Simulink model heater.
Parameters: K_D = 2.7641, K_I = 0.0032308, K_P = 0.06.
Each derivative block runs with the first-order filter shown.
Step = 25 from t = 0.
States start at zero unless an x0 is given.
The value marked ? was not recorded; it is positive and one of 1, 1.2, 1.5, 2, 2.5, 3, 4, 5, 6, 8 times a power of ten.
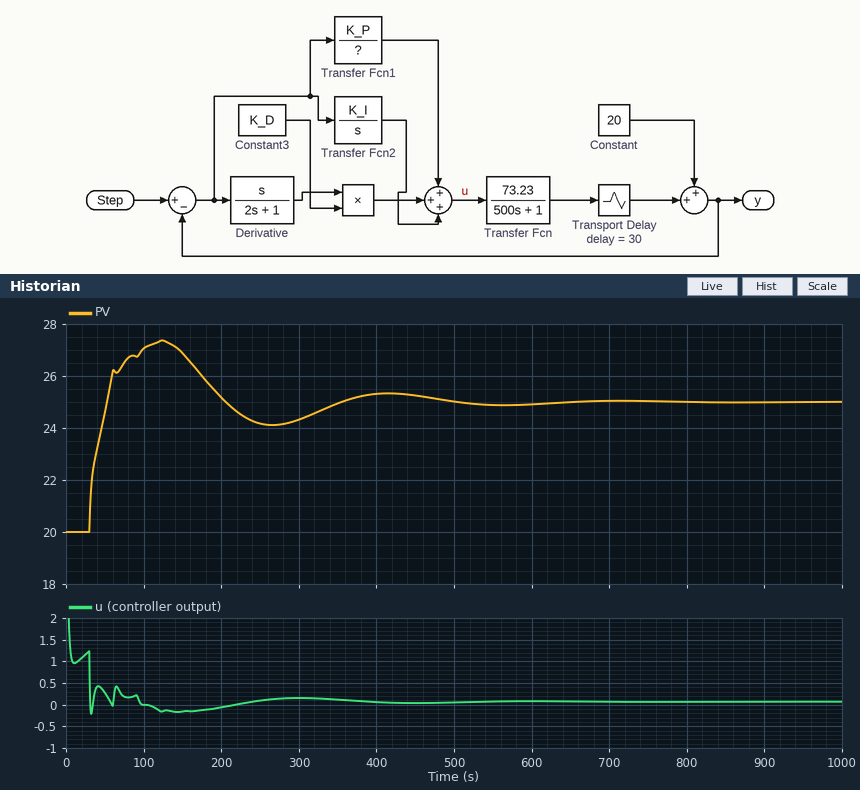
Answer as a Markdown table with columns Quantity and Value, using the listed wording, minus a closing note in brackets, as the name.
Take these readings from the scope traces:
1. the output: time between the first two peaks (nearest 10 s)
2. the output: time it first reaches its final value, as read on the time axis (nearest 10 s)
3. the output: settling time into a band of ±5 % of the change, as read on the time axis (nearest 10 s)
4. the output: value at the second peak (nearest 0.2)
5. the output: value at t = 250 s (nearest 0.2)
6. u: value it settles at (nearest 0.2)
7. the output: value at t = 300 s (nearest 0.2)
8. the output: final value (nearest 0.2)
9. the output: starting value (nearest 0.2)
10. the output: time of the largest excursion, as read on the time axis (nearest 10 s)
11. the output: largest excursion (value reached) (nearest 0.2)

| Quantity | Value |
|---|---|
| the output: time between the first two peaks | 290 s |
| the output: time it first reaches its final value, as read on the time axis | 50 s |
| the output: settling time into a band of ±5 % of the change, as read on the time axis | 450 s |
| the output: value at the second peak | 25.4 |
| the output: value at t = 250 s | 24.2 |
| u: value it settles at | 0.0 |
| the output: value at t = 300 s | 24.4 |
| the output: final value | 25.0 |
| the output: starting value | 20.0 |
| the output: time of the largest excursion, as read on the time axis | 120 s |
| the output: largest excursion (value reached) | 27.4 |
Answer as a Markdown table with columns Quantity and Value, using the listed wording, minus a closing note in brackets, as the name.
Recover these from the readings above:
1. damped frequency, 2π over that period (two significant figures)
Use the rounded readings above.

| Quantity | Value |
|---|---|
| damped frequency, 2π over that period | 0.022 rad/s |
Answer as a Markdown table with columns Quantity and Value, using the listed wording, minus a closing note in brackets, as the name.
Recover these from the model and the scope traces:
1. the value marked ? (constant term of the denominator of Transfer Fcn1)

| Quantity | Value |
|---|---|
| the value marked ? | 0.4 |
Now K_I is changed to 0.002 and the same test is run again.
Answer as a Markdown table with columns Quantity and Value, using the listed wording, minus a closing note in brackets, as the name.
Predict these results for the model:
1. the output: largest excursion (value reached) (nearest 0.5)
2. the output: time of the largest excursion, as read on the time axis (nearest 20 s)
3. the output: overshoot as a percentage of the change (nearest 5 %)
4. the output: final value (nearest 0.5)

| Quantity | Value |
|---|---|
| the output: largest excursion (value reached) | 26.5 |
| the output: time of the largest excursion, as read on the time axis | 140 s |
| the output: overshoot as a percentage of the change | 30 % |
| the output: final value | 25.0 |
